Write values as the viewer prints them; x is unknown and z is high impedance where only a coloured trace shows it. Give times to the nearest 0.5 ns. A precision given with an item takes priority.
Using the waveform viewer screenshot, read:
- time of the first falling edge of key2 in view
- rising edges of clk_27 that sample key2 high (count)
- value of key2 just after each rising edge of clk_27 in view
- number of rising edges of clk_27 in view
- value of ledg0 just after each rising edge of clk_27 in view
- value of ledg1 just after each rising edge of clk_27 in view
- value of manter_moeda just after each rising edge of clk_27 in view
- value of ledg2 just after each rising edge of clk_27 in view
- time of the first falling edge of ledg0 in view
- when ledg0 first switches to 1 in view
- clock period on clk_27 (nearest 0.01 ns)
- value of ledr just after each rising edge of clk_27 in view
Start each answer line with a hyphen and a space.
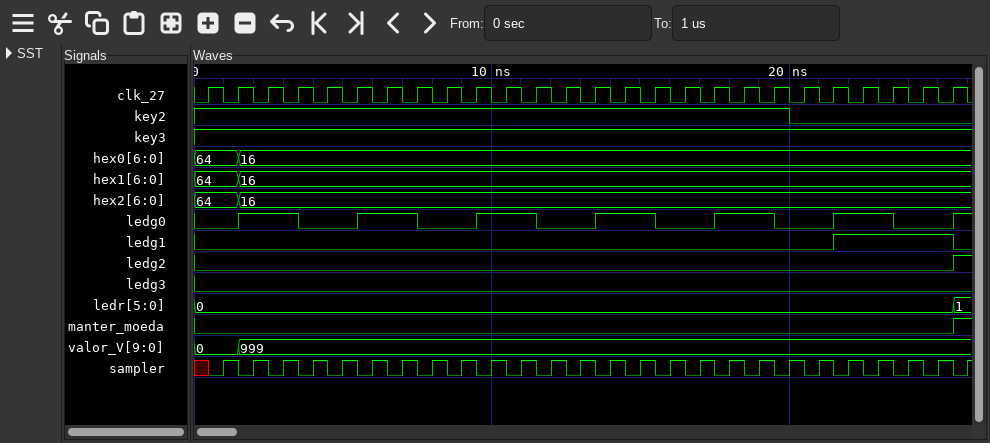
- 20 ns
- 20
- 1 1 1 1 1 1 1 1 1 1 1 1 1 1 1 1 1 1 1 1 0 0 0 0 0 0
- 26
- 0 1 1 0 0 1 1 0 0 1 1 0 0 1 1 0 0 1 1 0 0 1 1 0 0 1
- 0 0 0 0 0 0 0 0 0 0 0 0 0 0 0 0 0 0 0 0 0 1 1 1 1 0
- 0 0 0 0 0 0 0 0 0 0 0 0 0 0 0 0 0 0 0 0 0 0 0 0 0 1
- 0 0 0 0 0 0 0 0 0 0 0 0 0 0 0 0 0 0 0 0 0 0 0 0 0 1
- 3.5 ns
- 1.5 ns
- 1 ns
- 0, 0, 0, 0, 0, 0, 0, 0, 0, 0, 0, 0, 0, 0, 0, 0, 0, 0, 0, 0, 0, 0, 0, 0, 0, 1
